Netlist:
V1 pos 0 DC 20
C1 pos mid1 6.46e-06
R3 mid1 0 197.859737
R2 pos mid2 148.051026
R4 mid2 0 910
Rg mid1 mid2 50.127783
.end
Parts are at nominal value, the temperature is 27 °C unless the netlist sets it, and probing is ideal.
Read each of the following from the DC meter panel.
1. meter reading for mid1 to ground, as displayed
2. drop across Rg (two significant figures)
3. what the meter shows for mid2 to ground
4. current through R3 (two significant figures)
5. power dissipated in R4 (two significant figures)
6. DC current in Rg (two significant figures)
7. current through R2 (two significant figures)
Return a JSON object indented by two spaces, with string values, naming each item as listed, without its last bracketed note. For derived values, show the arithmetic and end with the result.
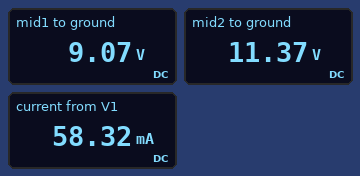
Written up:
{
  "meter reading for mid1 to ground, as displayed": "9.07 V",
  "drop across Rg": "11.37 V - 9.07 V = 2.3 V",
  "what the meter shows for mid2 to ground": "11.37 V",
  "current through R3": "(9.07 V) / 197.9 Ω = 46 mA",
  "power dissipated in R4": "(11.37 V)^2 / 910 Ω = 140 mW",
  "DC current in Rg": "(11.37 V - 9.07 V) / 50.13 Ω = 46 mA",
  "current through R2": "(20 V - 11.37 V) / 148.1 Ω = 58 mA"
}
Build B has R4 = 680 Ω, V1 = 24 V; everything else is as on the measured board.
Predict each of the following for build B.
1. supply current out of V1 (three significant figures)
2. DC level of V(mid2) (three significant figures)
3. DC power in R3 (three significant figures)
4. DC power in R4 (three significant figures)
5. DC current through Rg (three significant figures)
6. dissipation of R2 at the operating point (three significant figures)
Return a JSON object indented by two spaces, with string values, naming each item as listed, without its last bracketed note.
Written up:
{
  "supply current out of V1": "72.8 mA",
  "DC level of V(mid2)": "13.2 V",
  "DC power in R3": "563 mW",
  "DC power in R4": "257 mW",
  "DC current through Rg": "53.3 mA",
  "dissipation of R2 at the operating point": "784 mW"
}
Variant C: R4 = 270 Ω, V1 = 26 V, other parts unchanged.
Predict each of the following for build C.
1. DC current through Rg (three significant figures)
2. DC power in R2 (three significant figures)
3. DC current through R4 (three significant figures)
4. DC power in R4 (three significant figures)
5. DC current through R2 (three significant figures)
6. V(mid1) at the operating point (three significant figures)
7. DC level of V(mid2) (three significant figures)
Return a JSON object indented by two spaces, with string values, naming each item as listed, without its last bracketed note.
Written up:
{
  "DC current through Rg": "48.9 mA",
  "DC power in R2": "1.30 W",
  "DC current through R4": "44.9 mA",
  "DC power in R4": "544 mW",
  "DC current through R2": "93.8 mA",
  "V(mid1) at the operating point": "9.67 V",
  "DC level of V(mid2)": "12.1 V"
}
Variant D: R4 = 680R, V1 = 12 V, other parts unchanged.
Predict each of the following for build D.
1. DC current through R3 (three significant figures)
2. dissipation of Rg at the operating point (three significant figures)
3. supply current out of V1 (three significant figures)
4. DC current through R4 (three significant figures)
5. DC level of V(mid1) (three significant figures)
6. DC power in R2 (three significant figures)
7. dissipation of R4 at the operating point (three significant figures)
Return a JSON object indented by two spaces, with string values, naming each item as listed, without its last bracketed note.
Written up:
{
  "DC current through R3": "26.7 mA",
  "dissipation of Rg at the operating point": "35.6 mW",
  "supply current out of V1": "36.4 mA",
  "DC current through R4": "9.72 mA",
  "DC level of V(mid1)": "5.28 V",
  "DC power in R2": "196 mW",
  "dissipation of R4 at the operating point": "64.3 mW"
}
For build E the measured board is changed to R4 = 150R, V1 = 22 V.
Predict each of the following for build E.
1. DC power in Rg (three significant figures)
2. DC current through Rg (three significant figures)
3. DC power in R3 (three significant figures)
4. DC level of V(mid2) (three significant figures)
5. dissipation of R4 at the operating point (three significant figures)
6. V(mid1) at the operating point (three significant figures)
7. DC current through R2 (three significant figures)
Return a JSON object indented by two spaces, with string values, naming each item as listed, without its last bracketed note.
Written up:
{
  "DC power in Rg": "59.1 mW",
  "DC current through Rg": "34.3 mA",
  "DC power in R3": "233 mW",
  "DC level of V(mid2)": "8.51 V",
  "dissipation of R4 at the operating point": "483 mW",
  "V(mid1) at the operating point": "6.79 V",
  "DC current through R2": "91.1 mA"
}
